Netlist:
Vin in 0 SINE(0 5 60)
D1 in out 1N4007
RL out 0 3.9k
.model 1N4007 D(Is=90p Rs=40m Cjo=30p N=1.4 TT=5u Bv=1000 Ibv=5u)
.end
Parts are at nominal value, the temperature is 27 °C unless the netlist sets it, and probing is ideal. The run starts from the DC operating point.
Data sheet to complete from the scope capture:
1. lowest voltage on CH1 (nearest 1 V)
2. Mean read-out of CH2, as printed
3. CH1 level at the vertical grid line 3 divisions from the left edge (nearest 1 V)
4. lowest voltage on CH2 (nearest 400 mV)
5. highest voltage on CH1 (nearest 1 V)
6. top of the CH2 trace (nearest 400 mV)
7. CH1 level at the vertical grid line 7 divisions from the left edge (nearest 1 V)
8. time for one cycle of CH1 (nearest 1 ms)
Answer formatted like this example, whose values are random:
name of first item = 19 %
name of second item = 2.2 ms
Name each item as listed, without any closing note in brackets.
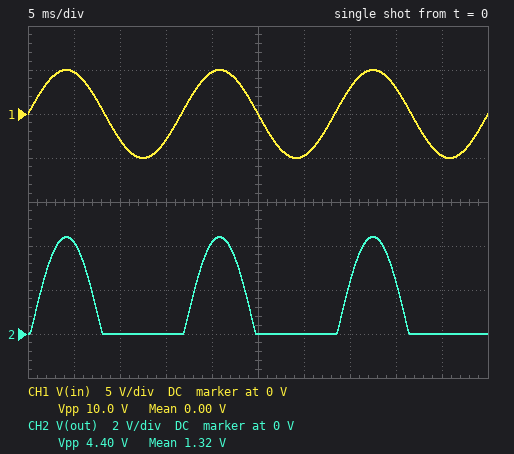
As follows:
lowest voltage on CH1 = -5 V
Mean read-out of CH2, as printed = 1.32 V
CH1 level at the vertical grid line 3 divisions from the left edge = -3 V
lowest voltage on CH2 = 0 V
highest voltage on CH1 = 5 V
top of the CH2 trace = 4.4 V
CH1 level at the vertical grid line 7 divisions from the left edge = 3 V
time for one cycle of CH1 = 17 ms
